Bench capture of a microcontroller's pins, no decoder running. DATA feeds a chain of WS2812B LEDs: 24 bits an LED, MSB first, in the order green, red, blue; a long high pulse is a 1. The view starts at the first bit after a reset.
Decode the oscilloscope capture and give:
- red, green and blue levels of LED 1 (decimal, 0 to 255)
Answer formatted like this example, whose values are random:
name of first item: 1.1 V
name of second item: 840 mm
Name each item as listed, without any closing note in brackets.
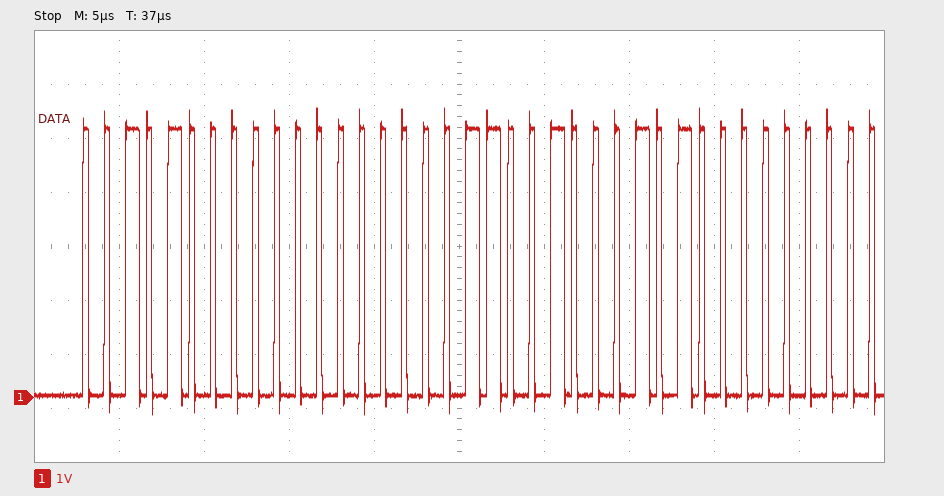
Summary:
red, green and blue levels of LED 1: 0, 40, 50
